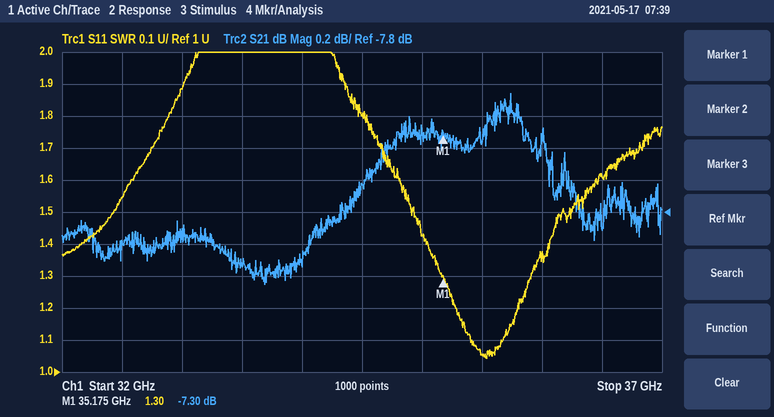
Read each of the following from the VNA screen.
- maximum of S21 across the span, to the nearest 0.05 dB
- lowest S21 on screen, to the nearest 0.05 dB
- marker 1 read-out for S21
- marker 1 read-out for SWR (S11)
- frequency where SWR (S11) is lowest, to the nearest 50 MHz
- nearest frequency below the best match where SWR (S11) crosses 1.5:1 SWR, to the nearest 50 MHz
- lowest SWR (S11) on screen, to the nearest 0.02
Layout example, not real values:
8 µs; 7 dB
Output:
-7.05 dB; -8.25 dB; -7.30 dB; 1.30; 35.55 GHz; 34.95 GHz; 1.04
